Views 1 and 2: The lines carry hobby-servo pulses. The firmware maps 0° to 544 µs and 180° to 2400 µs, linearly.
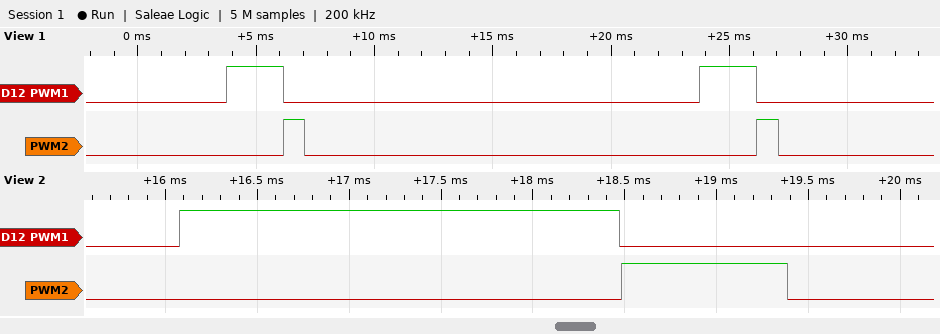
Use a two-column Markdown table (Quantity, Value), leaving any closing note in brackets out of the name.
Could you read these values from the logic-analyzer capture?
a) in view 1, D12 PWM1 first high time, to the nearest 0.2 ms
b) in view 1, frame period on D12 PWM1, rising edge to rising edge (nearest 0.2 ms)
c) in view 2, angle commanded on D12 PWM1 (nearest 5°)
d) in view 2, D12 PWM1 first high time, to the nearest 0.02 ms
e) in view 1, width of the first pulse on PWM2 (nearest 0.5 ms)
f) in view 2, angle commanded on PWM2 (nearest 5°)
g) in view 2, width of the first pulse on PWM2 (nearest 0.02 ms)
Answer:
| Quantity | Value |
|---|---|
| in view 1, D12 PWM1 first high time, to the nearest 0.2 ms | 2.4 ms |
| in view 1, frame period on D12 PWM1, rising edge to rising edge | 20.0 ms |
| in view 2, angle commanded on D12 PWM1 | 180° |
| in view 2, D12 PWM1 first high time, to the nearest 0.02 ms | 2.40 ms |
| in view 1, width of the first pulse on PWM2 | 1.0 ms |
| in view 2, angle commanded on PWM2 | 35° |
| in view 2, width of the first pulse on PWM2 | 0.90 ms |
